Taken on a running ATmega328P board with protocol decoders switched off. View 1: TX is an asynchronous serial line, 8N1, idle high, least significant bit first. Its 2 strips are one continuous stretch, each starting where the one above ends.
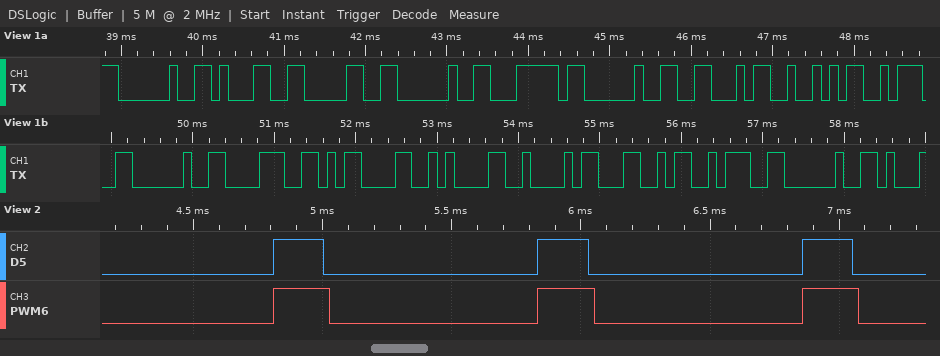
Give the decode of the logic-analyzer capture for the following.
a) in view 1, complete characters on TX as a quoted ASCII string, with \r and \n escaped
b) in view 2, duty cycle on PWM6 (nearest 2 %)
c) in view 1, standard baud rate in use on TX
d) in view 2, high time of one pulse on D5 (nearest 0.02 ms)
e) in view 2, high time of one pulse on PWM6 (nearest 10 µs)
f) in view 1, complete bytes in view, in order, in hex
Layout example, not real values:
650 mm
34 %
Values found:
" 10 | FR: 8\r\nBL: "
22 %
9600 baud
0.20 ms
220 µs
20 31 30 20 7C 20 46 52 3A 20 38 0D 0A 42 4C 3A 20
